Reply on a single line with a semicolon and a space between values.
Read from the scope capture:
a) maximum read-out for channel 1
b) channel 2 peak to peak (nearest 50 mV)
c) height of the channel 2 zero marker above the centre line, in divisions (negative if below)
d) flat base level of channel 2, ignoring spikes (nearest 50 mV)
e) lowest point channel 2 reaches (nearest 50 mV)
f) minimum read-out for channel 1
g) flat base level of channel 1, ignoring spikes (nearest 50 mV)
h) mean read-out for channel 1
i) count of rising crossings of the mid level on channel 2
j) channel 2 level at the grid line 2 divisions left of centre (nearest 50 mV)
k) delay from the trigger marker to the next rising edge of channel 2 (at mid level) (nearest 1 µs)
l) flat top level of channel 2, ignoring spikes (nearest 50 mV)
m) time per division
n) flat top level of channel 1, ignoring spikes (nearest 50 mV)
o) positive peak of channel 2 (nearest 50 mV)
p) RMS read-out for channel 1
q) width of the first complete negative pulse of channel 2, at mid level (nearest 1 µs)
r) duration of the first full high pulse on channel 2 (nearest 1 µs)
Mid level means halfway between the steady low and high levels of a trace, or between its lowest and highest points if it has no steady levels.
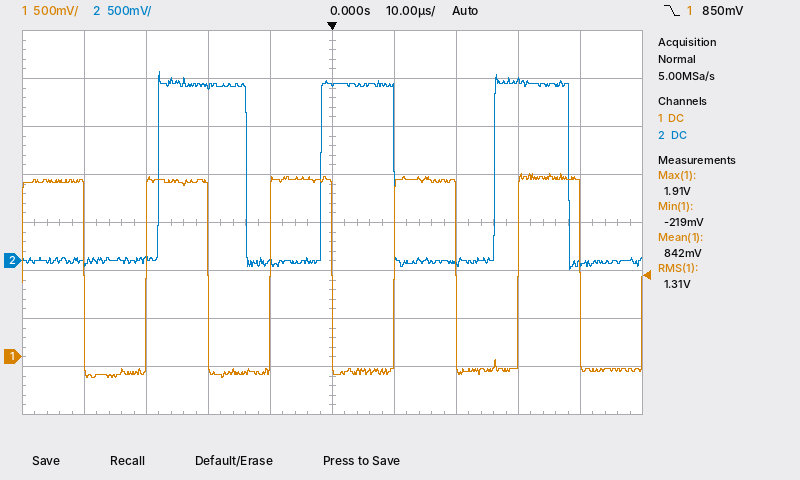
1.91 V; 2.05 V; -0.8 div; 0 mV; -100 mV; -219 mV; -150 mV; 842 mV; 3; 1.80 V; 26 µs; 1.85 V; 10 µs; 1.85 V; 1.95 V; 1.31 V; 12 µs; 14 µs
